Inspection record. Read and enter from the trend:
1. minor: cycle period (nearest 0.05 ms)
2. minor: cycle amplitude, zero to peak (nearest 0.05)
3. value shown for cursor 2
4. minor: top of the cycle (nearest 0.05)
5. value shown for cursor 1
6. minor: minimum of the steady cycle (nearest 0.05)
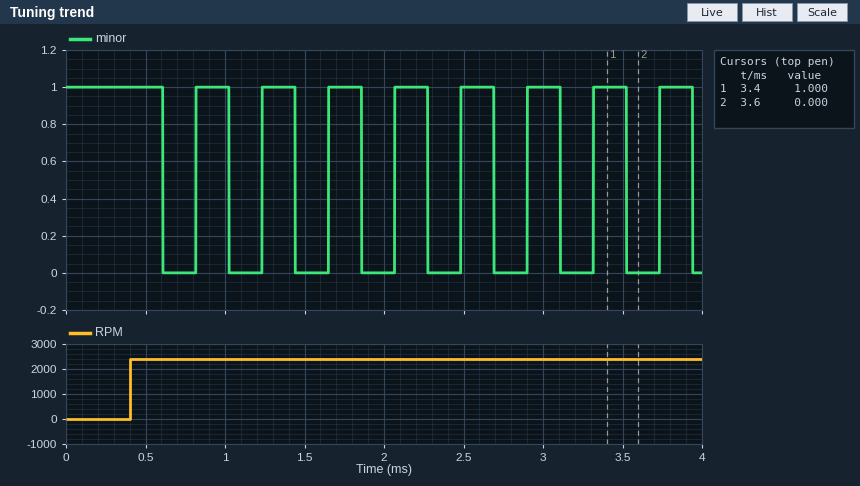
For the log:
0.40 ms
0.50
0.000
1.00
1.000
0.00
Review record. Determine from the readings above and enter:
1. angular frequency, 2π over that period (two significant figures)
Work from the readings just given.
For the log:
16 rad/ms
